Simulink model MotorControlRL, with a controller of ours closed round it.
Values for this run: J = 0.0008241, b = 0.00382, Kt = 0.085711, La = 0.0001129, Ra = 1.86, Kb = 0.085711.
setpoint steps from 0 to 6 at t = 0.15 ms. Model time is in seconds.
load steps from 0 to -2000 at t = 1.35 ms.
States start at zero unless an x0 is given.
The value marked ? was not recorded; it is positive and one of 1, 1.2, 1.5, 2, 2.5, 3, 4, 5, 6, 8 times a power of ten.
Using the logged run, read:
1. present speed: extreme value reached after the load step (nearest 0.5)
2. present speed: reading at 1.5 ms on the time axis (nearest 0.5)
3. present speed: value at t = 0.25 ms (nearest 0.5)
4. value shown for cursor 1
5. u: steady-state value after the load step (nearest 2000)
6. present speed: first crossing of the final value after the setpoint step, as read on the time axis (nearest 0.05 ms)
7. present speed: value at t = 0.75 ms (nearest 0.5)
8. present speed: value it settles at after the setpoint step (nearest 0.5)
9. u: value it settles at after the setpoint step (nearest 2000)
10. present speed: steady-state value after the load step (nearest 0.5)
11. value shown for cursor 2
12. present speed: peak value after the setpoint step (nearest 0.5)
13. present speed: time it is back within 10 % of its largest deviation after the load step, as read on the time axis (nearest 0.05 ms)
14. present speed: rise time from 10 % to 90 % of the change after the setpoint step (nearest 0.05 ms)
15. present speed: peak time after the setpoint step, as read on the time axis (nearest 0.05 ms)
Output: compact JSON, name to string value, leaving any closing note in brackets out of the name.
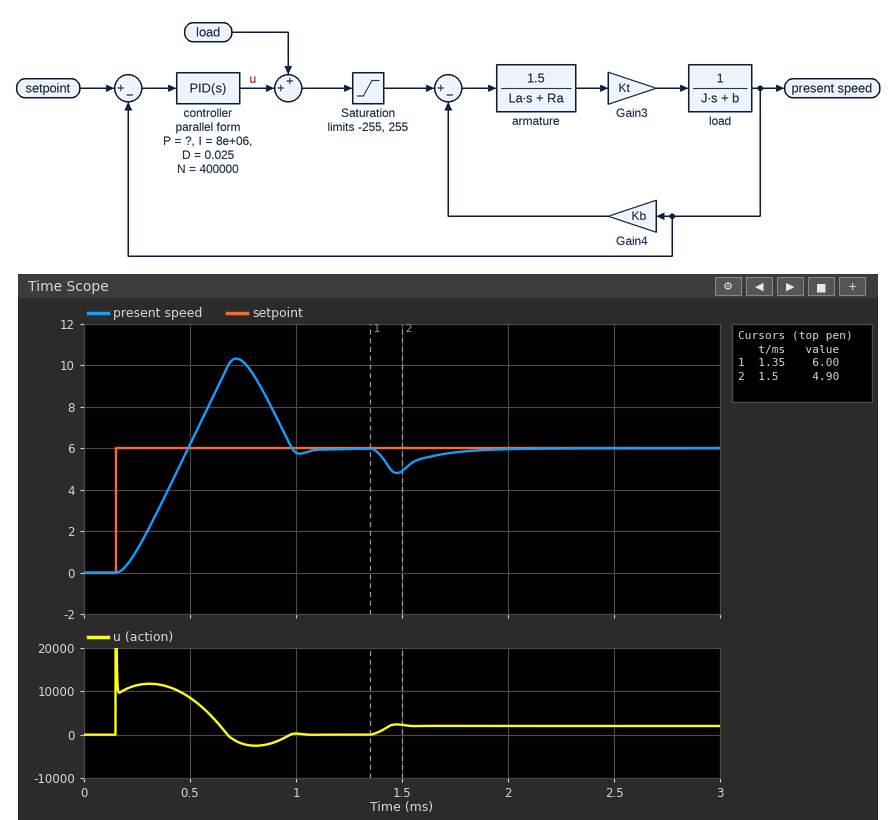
{"present speed: extreme value reached after the load step": "5.0", "present speed: reading at 1.5 ms on the time axis": "5.0", "present speed: value at t = 0.25 ms": "1.0", "value shown for cursor 1": "6.00", "u: steady-state value after the load step": "2000", "present speed: first crossing of the final value after the setpoint step, as read on the time axis": "0.50 ms", "present speed: value at t = 0.75 ms": "10.0", "present speed: value it settles at after the setpoint step": "6.0", "u: value it settles at after the setpoint step": "0", "present speed: steady-state value after the load step": "6.0", "value shown for cursor 2": "4.90", "present speed: peak value after the setpoint step": "10.5", "present speed: time it is back within 10 % of its largest deviation after the load step, as read on the time axis": "1.85 ms", "present speed: rise time from 10 % to 90 % of the change after the setpoint step": "0.25 ms", "present speed: peak time after the setpoint step, as read on the time axis": "0.70 ms"}
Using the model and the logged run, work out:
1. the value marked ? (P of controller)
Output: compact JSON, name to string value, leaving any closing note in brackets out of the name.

{"the value marked ?": "1500"}
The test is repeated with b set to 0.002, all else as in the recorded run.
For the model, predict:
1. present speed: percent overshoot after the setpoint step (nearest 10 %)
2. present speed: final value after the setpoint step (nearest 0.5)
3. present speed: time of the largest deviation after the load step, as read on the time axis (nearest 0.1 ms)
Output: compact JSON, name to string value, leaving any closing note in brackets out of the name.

{"present speed: percent overshoot after the setpoint step": "70 %", "present speed: final value after the setpoint step": "6.0", "present speed: time of the largest deviation after the load step, as read on the time axis": "1.5 ms"}
